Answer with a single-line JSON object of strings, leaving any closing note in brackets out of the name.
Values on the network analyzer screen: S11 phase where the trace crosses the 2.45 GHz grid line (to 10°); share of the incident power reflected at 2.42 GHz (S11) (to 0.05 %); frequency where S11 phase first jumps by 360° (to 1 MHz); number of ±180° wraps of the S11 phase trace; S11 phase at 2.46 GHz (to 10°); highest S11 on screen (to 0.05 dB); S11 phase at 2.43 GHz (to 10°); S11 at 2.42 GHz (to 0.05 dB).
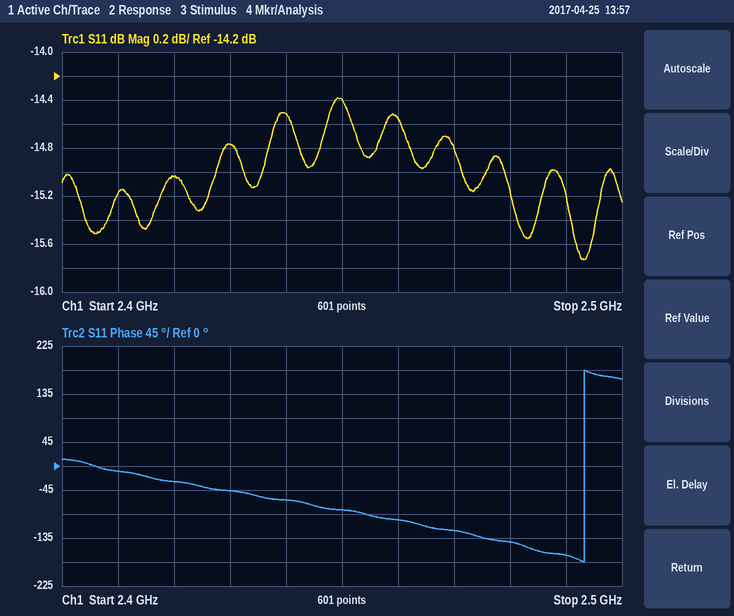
{"S11 phase where the trace crosses the 2.45 GHz grid line": "-80°", "share of the incident power reflected at 2.42 GHz (S11)": "3.15 %", "frequency where S11 phase first jumps by 360°": "2.493 GHz", "number of ±180° wraps of the S11 phase trace": "1", "S11 phase at 2.46 GHz": "-100°", "highest S11 on screen": "-14.40 dB", "S11 phase at 2.43 GHz": "-50°", "S11 at 2.42 GHz": "-15.05 dB"}
